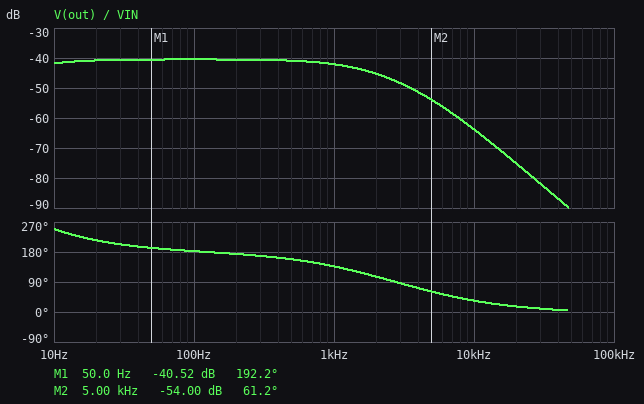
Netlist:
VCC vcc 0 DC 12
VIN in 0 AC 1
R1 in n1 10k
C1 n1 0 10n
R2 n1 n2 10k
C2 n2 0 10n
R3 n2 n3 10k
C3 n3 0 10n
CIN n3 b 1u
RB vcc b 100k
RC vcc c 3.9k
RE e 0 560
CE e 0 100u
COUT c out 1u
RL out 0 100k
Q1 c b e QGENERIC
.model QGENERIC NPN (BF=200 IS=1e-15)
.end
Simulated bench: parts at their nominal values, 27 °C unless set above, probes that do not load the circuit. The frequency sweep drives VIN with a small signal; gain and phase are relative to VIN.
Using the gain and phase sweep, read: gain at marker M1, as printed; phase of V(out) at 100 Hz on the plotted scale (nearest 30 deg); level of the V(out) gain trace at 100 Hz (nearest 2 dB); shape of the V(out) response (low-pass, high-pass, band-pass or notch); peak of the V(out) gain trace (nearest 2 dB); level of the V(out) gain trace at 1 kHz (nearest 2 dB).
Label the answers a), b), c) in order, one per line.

a) -40.52 dB
b) 180 deg
c) -40 dB
d) low-pass
e) -40 dB
f) -42 dB
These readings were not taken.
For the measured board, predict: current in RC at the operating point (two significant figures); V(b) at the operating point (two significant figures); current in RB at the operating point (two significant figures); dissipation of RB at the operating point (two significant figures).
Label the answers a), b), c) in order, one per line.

a) 2.7 mA
b) 2.3 V
c) 97 µA
d) 940 µW
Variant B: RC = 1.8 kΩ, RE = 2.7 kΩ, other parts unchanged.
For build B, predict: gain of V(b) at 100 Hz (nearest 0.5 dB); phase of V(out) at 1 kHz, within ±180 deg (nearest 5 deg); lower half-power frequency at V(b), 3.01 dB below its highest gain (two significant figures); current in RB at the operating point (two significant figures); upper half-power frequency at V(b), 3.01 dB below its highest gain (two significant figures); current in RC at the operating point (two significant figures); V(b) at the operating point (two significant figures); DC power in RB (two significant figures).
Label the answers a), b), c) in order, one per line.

a) -59.0 dB
b) 135 deg
c) 1.0 Hz
d) 41 µA
e) 7.9 Hz
f) 2.6 mA
g) 7.9 V
h) 170 µW
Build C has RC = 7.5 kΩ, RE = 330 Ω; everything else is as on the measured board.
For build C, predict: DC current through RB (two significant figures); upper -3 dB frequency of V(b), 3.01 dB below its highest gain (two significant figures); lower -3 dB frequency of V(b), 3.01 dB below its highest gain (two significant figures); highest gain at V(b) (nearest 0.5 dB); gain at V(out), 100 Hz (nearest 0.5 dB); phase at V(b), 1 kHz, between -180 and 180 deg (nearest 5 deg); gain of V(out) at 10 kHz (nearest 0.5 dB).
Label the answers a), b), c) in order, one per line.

a) 110 µA
b) 13 Hz
c) 2.1 Hz
d) -45.0 dB
e) -42.5 dB
f) -45 deg
g) -66.0 dB
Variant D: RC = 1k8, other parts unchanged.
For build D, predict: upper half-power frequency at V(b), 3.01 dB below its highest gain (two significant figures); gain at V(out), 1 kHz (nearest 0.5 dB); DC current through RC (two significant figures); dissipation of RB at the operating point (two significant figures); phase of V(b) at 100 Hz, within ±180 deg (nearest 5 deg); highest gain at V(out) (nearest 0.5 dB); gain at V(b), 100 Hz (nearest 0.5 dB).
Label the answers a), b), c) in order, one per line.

a) 11 Hz
b) -38.5 dB
c) 5.0 mA
d) 700 µW
e) -60 deg
f) -37.0 dB
g) -62.5 dB
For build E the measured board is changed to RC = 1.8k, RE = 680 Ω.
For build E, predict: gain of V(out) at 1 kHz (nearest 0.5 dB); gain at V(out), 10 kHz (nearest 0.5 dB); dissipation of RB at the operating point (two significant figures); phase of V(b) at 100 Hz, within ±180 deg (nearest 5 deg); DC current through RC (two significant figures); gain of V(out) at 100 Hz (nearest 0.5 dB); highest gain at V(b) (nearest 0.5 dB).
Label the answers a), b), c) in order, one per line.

a) -38.0 dB
b) -60.0 dB
c) 630 µW
d) -60 deg
e) 4.8 mA
f) -36.5 dB
g) -42.0 dB
